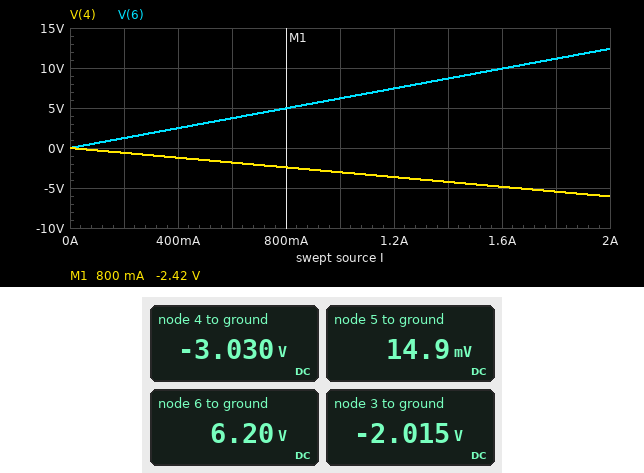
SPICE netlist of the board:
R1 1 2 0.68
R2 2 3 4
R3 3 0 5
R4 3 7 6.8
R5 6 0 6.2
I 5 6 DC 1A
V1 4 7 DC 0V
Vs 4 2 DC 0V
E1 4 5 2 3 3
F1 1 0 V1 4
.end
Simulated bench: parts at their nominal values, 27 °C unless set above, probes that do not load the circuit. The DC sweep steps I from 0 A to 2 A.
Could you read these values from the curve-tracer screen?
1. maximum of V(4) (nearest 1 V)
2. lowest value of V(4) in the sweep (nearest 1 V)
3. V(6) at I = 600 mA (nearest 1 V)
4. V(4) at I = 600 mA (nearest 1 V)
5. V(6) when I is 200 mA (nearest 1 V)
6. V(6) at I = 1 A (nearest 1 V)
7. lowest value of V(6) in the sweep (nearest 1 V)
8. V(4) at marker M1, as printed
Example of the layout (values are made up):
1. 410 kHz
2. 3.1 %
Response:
1. 0 V
2. -6 V
3. 4 V
4. -2 V
5. 1 V
6. 6 V
7. 0 V
8. -2.42 V
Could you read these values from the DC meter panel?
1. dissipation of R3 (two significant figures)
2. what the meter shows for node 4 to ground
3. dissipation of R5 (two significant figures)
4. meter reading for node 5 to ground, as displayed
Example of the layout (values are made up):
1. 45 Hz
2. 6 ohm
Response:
1. 810 mW
2. -3.030 V
3. 6.2 W
4. 14.9 mV
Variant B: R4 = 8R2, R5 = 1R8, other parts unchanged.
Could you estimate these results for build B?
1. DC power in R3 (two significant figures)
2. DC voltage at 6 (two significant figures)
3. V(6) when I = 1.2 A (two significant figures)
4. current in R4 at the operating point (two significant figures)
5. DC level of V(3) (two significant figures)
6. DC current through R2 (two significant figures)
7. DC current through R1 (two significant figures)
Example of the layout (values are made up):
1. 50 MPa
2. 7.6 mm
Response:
1. 940 mW
2. 1.8 V
3. 2.2 V
4. 140 mA
5. -2.2 V
6. 290 mA
7. 570 mA
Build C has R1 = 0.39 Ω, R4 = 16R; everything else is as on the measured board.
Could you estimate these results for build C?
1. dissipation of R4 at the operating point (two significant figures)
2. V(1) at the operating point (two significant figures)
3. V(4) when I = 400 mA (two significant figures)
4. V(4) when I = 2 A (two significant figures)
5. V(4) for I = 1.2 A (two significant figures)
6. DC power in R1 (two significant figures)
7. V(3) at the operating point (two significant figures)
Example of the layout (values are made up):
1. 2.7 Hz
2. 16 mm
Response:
1. 200 mW
2. -4.4 V
3. -1.8 V
4. -9.1 V
5. -5.5 V
6. 77 mW
7. -2.8 V
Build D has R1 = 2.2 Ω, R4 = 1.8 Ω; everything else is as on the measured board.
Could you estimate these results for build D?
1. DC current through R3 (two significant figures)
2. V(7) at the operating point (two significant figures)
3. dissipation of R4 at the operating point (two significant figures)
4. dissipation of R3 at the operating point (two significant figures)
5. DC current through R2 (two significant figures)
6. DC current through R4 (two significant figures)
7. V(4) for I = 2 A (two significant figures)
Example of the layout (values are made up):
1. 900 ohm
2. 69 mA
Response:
1. 270 mA
2. -1.7 V
3. 61 mW
4. 350 mW
5. 83 mA
6. 180 mA
7. -3.3 V
